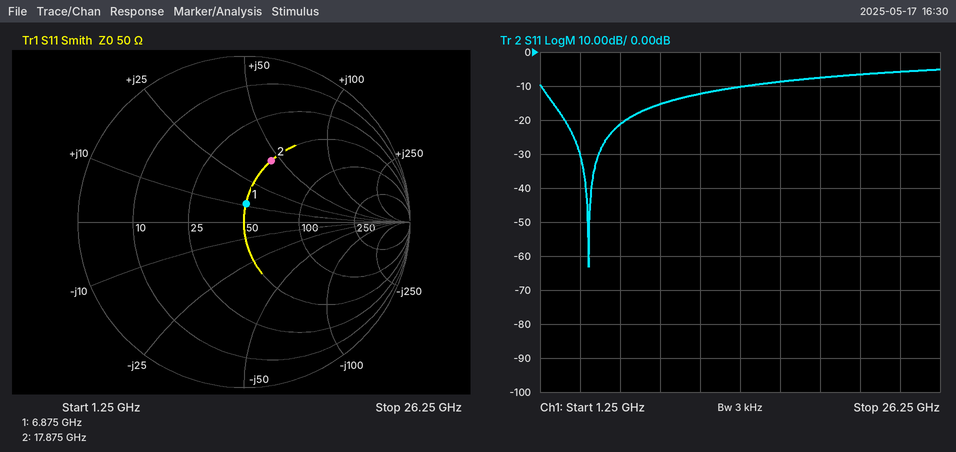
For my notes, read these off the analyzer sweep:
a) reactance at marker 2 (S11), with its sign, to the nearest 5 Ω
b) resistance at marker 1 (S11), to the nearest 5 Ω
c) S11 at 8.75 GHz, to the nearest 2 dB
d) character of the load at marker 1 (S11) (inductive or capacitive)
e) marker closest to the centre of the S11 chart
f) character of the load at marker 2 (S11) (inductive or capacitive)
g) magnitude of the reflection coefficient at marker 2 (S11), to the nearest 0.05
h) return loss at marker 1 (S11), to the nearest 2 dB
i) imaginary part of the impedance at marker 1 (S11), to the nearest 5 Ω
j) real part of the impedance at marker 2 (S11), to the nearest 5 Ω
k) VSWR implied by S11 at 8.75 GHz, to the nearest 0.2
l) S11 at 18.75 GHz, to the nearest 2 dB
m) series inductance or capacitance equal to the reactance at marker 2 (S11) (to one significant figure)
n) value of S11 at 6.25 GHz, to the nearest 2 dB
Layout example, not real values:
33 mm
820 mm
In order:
+45 Ω
50 Ω
-16 dB
inductive
marker 1
inductive
0.40
20 dB
+10 Ω
50 Ω
1.4
-8 dB
400 pH
-22 dB
